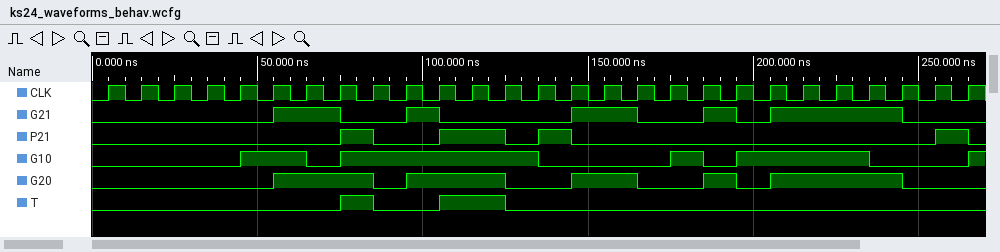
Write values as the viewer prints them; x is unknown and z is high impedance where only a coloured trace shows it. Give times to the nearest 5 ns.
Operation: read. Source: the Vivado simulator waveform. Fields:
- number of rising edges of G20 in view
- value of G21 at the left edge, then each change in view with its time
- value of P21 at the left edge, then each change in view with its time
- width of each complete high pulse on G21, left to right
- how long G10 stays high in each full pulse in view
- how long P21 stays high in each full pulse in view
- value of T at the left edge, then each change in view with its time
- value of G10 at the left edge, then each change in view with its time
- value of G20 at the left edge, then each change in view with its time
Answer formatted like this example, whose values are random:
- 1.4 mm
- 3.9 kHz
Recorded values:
- 5
- 0, 1 at 55 ns, 0 at 75 ns, 1 at 95 ns, 0 at 105 ns, 1 at 145 ns, 0 at 165 ns, 1 at 185 ns, 0 at 195 ns, 1 at 205 ns, 0 at 245 ns
- 0, 1 at 75 ns, 0 at 85 ns, 1 at 105 ns, 0 at 125 ns, 1 at 135 ns, 0 at 145 ns, 1 at 255 ns, 0 at 265 ns
- 20 ns, 10 ns, 20 ns, 10 ns, 40 ns
- 20 ns, 60 ns, 10 ns, 40 ns
- 10 ns, 20 ns, 10 ns, 10 ns
- 0, 1 at 75 ns, 0 at 85 ns, 1 at 105 ns, 0 at 125 ns
- 0, 1 at 45 ns, 0 at 65 ns, 1 at 75 ns, 0 at 135 ns, 1 at 175 ns, 0 at 185 ns, 1 at 195 ns, 0 at 235 ns, 1 at 265 ns
- 0, 1 at 55 ns, 0 at 85 ns, 1 at 95 ns, 0 at 125 ns, 1 at 145 ns, 0 at 165 ns, 1 at 185 ns, 0 at 195 ns, 1 at 205 ns, 0 at 245 ns
